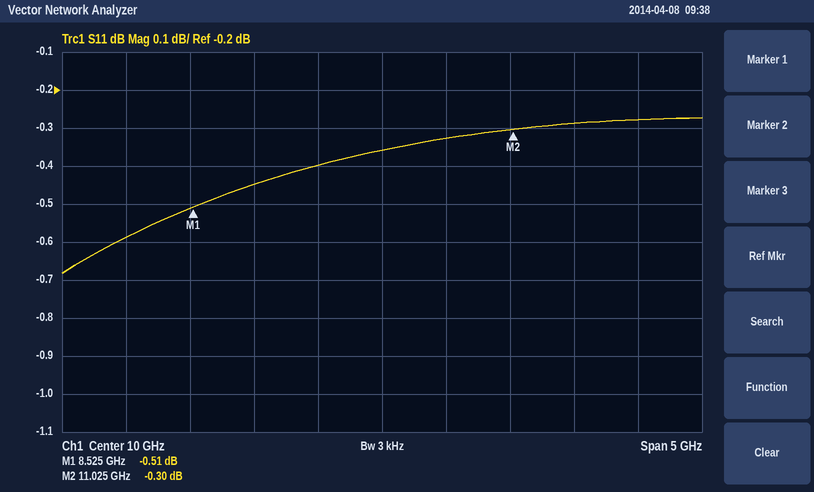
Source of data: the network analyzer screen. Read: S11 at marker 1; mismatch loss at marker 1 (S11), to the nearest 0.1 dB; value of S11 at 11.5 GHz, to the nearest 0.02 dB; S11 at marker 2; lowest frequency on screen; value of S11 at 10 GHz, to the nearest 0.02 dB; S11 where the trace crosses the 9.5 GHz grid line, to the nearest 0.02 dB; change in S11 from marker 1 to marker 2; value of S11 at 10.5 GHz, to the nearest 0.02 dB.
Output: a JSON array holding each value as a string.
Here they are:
["-0.51 dB", "9.6 dB", "-0.28 dB", "-0.30 dB", "7.5 GHz", "-0.36 dB", "-0.40 dB", "0.21 dB", "-0.32 dB"]
